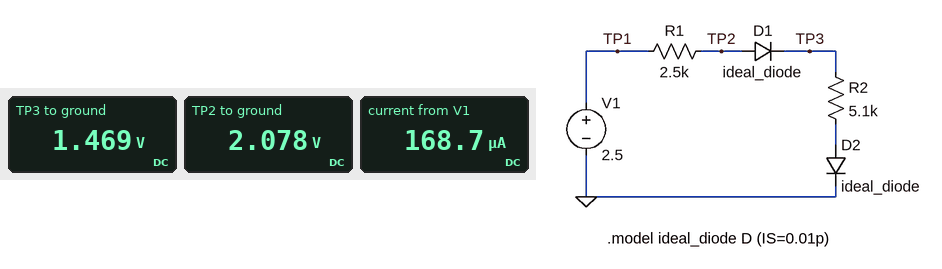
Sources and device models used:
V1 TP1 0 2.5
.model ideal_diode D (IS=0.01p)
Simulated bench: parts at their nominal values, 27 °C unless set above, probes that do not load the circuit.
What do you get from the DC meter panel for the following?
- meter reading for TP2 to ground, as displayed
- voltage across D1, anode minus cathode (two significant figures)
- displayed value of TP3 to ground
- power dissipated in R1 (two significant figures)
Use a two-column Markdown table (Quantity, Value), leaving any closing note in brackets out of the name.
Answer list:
| Quantity | Value |
|---|---|
| meter reading for TP2 to ground, as displayed | 2.078 V |
| voltage across D1, anode minus cathode | 610 mV |
| displayed value of TP3 to ground | 1.469 V |
| power dissipated in R1 | 71 µW |
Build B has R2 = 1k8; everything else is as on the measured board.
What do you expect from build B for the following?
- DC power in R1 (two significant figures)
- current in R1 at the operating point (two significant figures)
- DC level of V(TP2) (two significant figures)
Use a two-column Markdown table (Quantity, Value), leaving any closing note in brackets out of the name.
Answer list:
| Quantity | Value |
|---|---|
| DC power in R1 | 210 µW |
| current in R1 at the operating point | 290 µA |
| DC level of V(TP2) | 1.8 V |
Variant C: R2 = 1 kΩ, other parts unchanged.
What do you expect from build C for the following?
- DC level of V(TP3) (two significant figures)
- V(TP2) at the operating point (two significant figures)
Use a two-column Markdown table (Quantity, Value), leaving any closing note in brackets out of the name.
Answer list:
| Quantity | Value |
|---|---|
| DC level of V(TP3) | 980 mV |
| V(TP2) at the operating point | 1.6 V |
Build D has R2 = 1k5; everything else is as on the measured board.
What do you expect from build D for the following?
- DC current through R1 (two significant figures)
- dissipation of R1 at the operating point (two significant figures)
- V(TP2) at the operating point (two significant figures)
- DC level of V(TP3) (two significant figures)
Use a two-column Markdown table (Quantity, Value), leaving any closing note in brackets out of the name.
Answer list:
| Quantity | Value |
|---|---|
| DC current through R1 | 310 µA |
| dissipation of R1 at the operating point | 240 µW |
| V(TP2) at the operating point | 1.7 V |
| DC level of V(TP3) | 1.1 V |
